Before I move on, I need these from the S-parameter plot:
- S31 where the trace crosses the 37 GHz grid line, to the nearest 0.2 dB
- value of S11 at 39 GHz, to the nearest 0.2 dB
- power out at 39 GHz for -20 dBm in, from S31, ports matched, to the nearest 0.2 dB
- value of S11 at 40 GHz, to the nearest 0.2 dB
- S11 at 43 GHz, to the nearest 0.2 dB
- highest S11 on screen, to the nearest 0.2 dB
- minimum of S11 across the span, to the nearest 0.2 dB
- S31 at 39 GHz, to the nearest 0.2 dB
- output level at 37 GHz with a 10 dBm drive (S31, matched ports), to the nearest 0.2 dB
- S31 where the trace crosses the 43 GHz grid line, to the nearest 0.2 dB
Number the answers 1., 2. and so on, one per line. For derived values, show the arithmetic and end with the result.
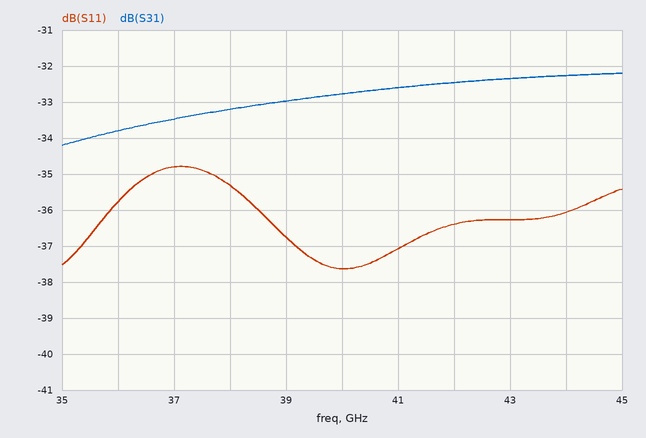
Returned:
1. -33.4 dB
2. -36.8 dB
3. -20 dBm + (-33.0 dB) = -53.0 dBm
4. -37.6 dB
5. -36.2 dB
6. -34.8 dB
7. -37.6 dB
8. -33.0 dB
9. 10 dBm + (-33.4 dB) = -23.4 dBm
10. -32.4 dB
